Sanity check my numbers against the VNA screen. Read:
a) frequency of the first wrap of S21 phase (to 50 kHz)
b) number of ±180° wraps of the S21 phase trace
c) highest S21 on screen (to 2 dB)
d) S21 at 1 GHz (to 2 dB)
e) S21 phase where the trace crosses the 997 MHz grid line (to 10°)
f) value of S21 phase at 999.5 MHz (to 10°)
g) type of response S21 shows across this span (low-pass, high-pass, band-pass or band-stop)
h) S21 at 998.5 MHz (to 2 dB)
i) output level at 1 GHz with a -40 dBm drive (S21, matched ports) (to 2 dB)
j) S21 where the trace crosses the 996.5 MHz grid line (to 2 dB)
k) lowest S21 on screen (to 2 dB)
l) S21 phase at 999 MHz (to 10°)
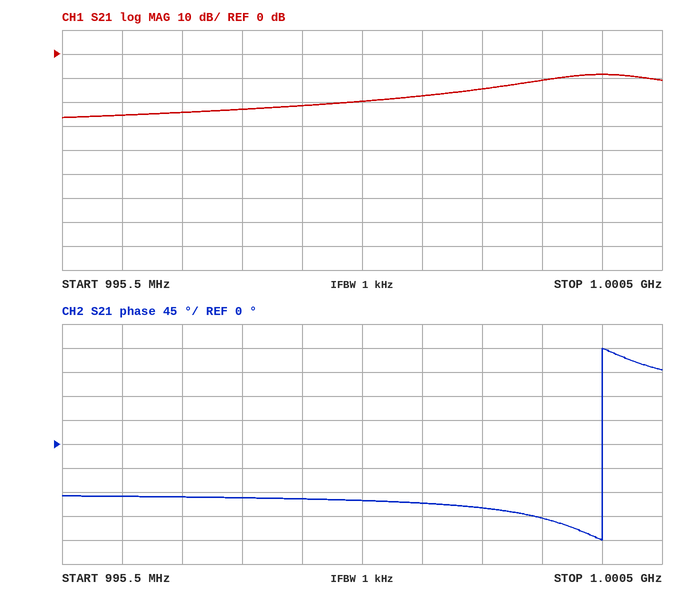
1.00000 GHz
1
-8 dB
-8 dB
-100°
-140°
high-pass
-18 dB
-48 dBm
-24 dB
-26 dB
-120°
